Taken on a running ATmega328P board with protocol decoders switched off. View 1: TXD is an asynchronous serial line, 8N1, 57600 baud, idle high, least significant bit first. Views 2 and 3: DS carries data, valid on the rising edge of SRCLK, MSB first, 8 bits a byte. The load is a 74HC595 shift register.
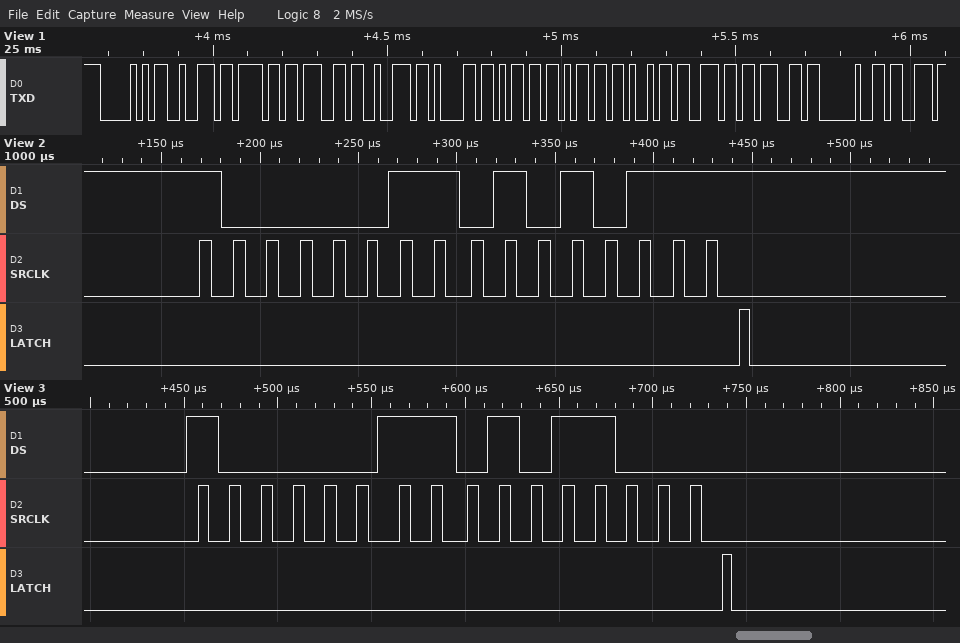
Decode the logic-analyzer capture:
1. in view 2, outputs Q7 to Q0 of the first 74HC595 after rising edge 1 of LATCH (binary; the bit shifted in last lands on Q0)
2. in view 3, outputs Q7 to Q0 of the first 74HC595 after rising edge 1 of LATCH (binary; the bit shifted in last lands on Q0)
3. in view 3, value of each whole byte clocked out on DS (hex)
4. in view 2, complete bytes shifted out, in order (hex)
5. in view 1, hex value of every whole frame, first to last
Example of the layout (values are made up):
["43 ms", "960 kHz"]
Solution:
["01010111", "01011000", "0x83 0x58", "83 57", "50 72 6F 67 72 61 6D 6D 69 6E 67 20 73"]
